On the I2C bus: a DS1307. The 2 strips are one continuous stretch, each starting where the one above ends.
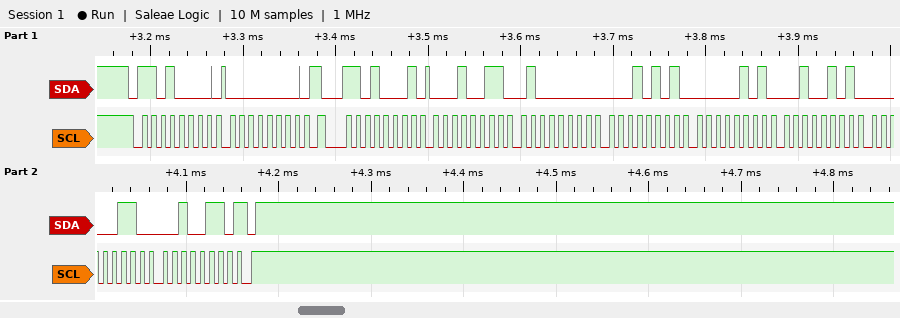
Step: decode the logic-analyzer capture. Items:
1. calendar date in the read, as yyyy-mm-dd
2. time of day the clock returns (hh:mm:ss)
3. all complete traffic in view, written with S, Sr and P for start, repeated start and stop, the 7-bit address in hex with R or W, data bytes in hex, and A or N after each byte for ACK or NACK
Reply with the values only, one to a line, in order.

2026-06-25
15:40:13
S 68W A 00 A Sr 68R A 13 A 40 A 15 A 05 A 25 A 06 A 26 N P
